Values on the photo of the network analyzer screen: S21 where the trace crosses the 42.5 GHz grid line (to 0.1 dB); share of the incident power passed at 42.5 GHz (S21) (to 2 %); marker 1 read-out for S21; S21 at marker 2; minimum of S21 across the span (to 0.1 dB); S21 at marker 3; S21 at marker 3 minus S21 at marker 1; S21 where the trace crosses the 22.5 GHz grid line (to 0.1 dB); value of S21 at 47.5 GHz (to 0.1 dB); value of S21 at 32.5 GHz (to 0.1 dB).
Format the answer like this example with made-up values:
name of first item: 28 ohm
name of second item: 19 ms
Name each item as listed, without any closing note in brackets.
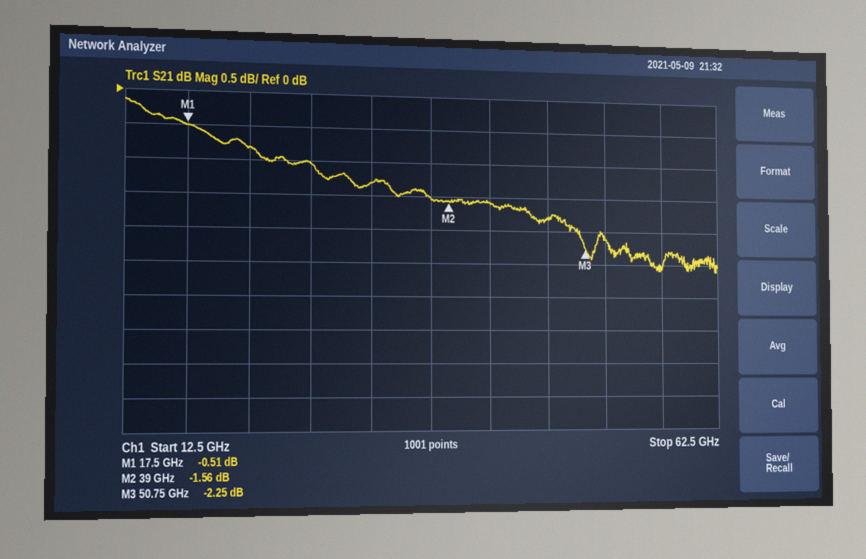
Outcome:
S21 where the trace crosses the 42.5 GHz grid line: -1.6 dB
share of the incident power passed at 42.5 GHz (S21): 70 %
marker 1 read-out for S21: -0.51 dB
S21 at marker 2: -1.56 dB
minimum of S21 across the span: -2.6 dB
S21 at marker 3: -2.25 dB
S21 at marker 3 minus S21 at marker 1: -1.74 dB
S21 where the trace crosses the 22.5 GHz grid line: -0.8 dB
value of S21 at 47.5 GHz: -1.8 dB
value of S21 at 32.5 GHz: -1.3 dB
